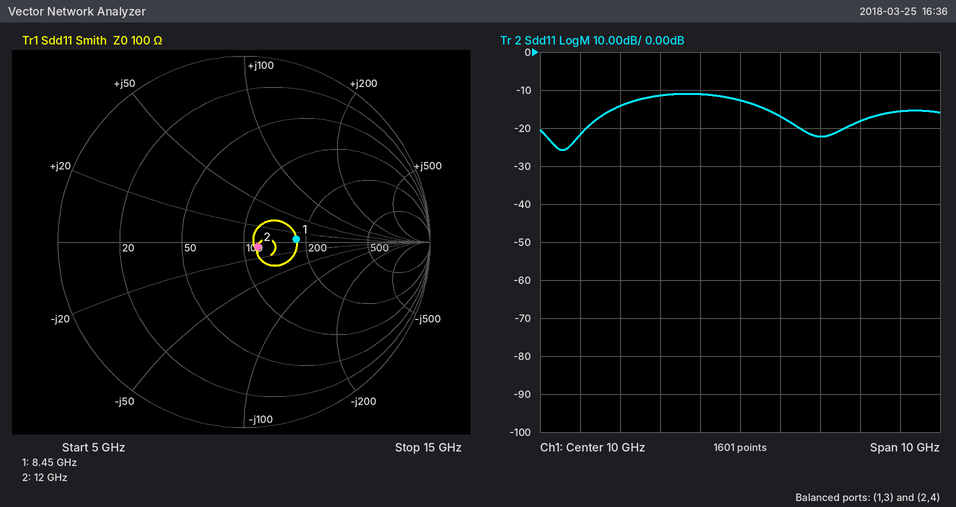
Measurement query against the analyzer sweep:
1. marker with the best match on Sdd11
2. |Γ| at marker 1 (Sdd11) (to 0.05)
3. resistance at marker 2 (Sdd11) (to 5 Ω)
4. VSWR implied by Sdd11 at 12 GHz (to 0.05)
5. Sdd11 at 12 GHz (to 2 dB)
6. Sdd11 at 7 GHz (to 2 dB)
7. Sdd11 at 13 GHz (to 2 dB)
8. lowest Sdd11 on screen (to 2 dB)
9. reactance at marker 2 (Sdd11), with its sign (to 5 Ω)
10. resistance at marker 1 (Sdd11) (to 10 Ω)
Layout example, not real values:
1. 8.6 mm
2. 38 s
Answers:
1. marker 2
2. 0.30
3. 115 Ω
4. 1.15
5. -22 dB
6. -14 dB
7. -18 dB
8. -26 dB
9. -5 Ω
10. 180 Ω
